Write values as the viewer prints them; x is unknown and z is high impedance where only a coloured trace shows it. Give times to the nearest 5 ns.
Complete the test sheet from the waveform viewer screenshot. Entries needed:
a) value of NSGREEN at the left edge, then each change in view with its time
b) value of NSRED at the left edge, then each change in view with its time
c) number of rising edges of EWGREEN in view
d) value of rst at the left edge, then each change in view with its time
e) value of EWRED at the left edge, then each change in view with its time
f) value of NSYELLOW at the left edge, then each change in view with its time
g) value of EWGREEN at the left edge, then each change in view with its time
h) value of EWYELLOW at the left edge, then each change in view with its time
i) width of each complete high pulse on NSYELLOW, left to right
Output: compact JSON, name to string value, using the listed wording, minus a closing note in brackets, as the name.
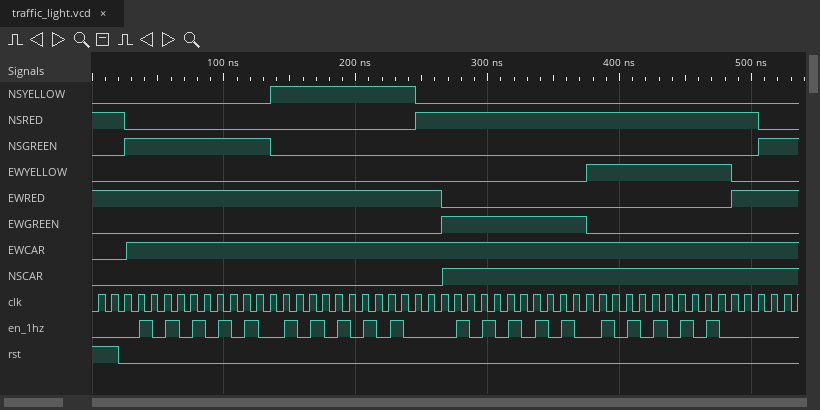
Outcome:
{"value of NSGREEN at the left edge, then each change in view with its time": "0, 1 at 25 ns, 0 at 135 ns, 1 at 505 ns", "value of NSRED at the left edge, then each change in view with its time": "1, 0 at 25 ns, 1 at 245 ns, 0 at 505 ns", "number of rising edges of EWGREEN in view": "1", "value of rst at the left edge, then each change in view with its time": "1, 0 at 20 ns", "value of EWRED at the left edge, then each change in view with its time": "1, 0 at 265 ns, 1 at 485 ns", "value of NSYELLOW at the left edge, then each change in view with its time": "0, 1 at 135 ns, 0 at 245 ns", "value of EWGREEN at the left edge, then each change in view with its time": "0, 1 at 265 ns, 0 at 375 ns", "value of EWYELLOW at the left edge, then each change in view with its time": "0, 1 at 375 ns, 0 at 485 ns", "width of each complete high pulse on NSYELLOW, left to right": "110 ns"}
